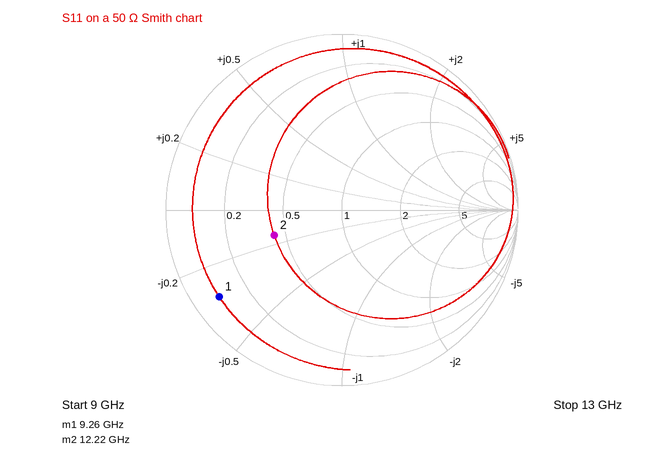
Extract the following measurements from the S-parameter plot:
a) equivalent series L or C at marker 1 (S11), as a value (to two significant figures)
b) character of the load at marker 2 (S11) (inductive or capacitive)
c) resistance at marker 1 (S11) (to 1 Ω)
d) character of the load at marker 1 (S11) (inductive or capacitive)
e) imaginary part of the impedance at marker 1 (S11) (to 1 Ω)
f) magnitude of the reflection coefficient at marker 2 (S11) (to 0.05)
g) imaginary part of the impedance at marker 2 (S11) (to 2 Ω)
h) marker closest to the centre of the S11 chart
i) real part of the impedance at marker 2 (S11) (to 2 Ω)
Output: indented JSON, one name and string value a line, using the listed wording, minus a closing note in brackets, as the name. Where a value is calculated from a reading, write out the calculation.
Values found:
{
  "equivalent series L or C at marker 1 (S11), as a value": "C = 1/(2π × 9.26 GHz × 16 Ω) ≈ 1.1 pF",
  "character of the load at marker 2 (S11)": "capacitive",
  "resistance at marker 1 (S11)": "4 Ω",
  "character of the load at marker 1 (S11)": "capacitive",
  "imaginary part of the impedance at marker 1 (S11)": "-16 Ω",
  "magnitude of the reflection coefficient at marker 2 (S11)": "0.40",
  "imaginary part of the impedance at marker 2 (S11)": "-8 Ω",
  "marker closest to the centre of the S11 chart": "marker 2",
  "real part of the impedance at marker 2 (S11)": "22 Ω"
}
